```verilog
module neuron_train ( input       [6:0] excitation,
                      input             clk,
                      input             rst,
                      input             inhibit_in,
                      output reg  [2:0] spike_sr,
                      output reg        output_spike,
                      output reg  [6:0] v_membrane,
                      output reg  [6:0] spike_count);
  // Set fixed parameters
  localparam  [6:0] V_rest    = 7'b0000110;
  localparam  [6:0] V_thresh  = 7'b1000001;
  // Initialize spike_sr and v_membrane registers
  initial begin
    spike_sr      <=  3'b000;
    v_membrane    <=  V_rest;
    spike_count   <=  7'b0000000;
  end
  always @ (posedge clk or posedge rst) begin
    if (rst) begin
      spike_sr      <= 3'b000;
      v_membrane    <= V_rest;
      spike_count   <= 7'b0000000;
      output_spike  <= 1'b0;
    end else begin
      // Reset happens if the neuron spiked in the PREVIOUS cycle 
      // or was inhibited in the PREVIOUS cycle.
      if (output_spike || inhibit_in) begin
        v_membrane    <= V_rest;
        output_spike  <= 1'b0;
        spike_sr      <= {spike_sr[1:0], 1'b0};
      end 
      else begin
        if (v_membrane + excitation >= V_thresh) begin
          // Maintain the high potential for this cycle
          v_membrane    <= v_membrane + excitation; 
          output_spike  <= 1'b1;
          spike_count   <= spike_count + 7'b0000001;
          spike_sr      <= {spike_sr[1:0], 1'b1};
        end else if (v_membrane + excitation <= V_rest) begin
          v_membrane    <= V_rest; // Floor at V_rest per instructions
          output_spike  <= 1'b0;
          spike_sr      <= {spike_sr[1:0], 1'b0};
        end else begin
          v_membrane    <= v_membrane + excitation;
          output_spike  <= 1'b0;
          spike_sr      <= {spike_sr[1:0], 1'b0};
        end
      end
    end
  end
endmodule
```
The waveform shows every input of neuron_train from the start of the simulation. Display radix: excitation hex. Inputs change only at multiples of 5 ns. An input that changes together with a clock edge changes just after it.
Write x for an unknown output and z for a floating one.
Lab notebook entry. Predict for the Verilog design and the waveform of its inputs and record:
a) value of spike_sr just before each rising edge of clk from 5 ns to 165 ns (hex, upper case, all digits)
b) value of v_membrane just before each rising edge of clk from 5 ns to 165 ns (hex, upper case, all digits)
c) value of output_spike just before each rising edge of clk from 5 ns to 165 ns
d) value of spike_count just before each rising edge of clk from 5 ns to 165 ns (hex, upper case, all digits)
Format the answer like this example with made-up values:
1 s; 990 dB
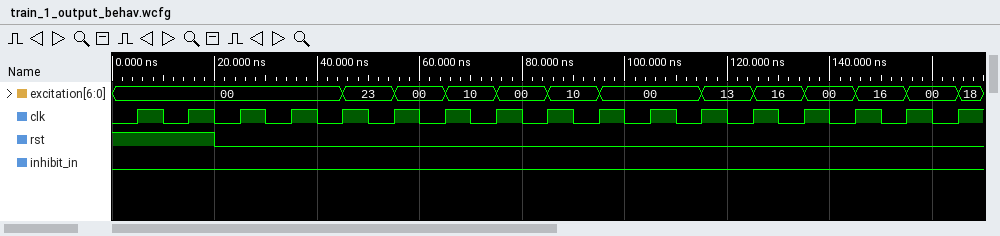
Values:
0, 0, 0, 0, 0, 0, 0, 0, 0, 0, 1, 2, 4, 0, 0, 0, 1; 06, 06, 06, 06, 06, 06, 29, 29, 39, 39, 49, 06, 06, 19, 2F, 2F, 45; 0 0 0 0 0 0 0 0 0 0 1 0 0 0 0 0 1; 00, 00, 00, 00, 00, 00, 00, 00, 00, 00, 01, 01, 01, 01, 01, 01, 02
